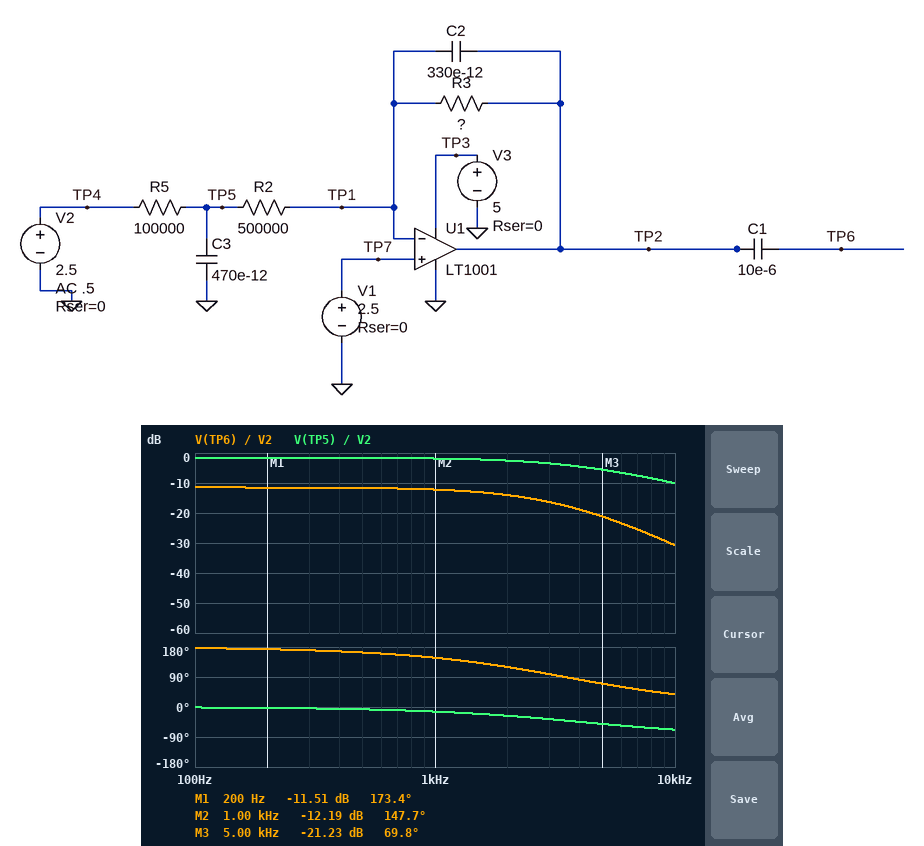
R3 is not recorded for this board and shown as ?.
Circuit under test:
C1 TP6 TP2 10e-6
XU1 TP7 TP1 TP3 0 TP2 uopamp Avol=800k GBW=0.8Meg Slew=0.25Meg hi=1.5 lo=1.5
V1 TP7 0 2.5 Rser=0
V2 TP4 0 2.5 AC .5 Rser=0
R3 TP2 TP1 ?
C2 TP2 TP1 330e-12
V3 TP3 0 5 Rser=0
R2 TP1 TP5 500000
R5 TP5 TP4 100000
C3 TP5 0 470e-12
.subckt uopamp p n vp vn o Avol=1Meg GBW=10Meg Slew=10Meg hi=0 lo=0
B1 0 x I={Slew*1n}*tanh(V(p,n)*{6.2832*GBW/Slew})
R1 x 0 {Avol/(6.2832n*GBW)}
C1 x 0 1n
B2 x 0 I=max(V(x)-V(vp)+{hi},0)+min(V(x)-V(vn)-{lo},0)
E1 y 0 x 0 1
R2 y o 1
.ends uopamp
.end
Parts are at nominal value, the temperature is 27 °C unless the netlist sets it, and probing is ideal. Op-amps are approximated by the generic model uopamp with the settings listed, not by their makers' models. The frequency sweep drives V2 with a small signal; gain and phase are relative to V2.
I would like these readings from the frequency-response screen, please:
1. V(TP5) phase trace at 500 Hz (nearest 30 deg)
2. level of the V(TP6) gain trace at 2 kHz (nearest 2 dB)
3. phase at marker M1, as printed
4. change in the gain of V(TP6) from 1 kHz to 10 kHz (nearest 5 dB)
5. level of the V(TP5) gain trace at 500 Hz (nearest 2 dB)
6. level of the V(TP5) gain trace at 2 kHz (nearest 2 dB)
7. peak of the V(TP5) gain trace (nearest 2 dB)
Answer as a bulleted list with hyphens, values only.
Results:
- 0 deg
- -14 dB
- 173.4 deg
- -20 dB
- -2 dB
- -2 dB
- -2 dB
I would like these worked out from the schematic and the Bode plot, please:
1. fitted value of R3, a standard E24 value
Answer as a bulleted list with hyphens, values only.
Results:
- 160 kΩ
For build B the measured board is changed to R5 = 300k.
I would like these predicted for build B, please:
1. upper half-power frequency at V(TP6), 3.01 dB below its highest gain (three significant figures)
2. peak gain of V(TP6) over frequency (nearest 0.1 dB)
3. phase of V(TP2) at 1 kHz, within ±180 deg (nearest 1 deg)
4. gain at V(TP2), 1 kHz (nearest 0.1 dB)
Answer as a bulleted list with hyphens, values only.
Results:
- 1.43 kHz
- -14.0 dB
- 133 deg
- -15.6 dB
